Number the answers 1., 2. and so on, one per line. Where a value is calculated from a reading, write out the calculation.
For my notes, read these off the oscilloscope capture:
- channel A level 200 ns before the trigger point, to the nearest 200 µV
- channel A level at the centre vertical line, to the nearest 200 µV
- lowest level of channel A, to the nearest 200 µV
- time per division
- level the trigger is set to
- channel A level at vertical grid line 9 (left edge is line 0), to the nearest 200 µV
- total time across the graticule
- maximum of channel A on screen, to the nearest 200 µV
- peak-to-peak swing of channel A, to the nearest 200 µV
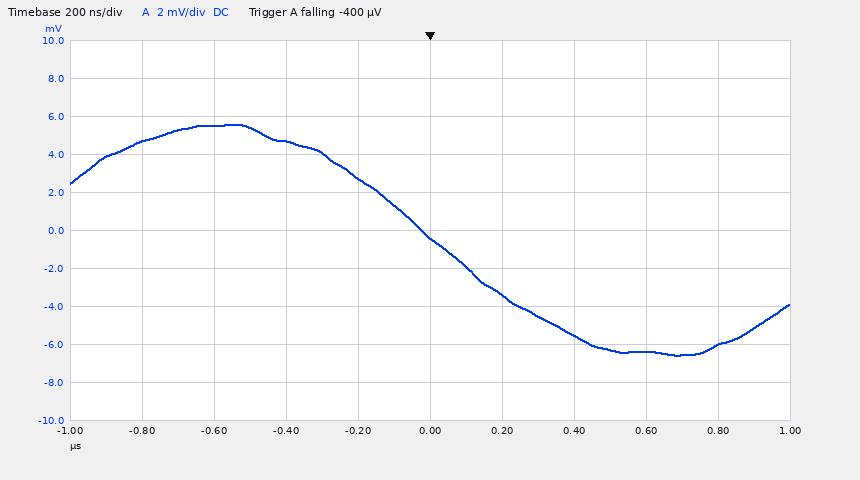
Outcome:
1. 2.8 mV
2. -400 µV
3. -6.6 mV
4. 200 ns
5. -400 µV
6. -6.0 mV
7. 2 µs
8. 5.6 mV
9. 5.6 mV − (-6.6 mV) = 12.2 mV
